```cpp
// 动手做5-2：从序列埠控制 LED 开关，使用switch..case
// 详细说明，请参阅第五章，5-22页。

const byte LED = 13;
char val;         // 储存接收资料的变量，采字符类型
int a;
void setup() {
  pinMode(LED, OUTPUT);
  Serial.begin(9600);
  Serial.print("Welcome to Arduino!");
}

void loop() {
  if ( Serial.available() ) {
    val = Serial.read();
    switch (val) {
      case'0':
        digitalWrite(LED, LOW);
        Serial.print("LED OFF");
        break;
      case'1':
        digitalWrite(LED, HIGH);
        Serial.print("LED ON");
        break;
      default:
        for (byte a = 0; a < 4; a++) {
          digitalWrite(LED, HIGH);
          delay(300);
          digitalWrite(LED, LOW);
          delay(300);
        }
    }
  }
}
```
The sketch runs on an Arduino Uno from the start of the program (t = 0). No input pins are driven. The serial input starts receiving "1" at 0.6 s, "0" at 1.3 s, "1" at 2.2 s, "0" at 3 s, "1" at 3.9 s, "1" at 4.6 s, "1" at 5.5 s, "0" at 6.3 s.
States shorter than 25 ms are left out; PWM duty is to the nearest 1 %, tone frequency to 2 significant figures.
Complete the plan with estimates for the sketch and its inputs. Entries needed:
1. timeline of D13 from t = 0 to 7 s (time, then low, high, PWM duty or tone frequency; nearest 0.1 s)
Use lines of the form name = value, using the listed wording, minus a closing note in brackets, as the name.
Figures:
timeline of D13 from t = 0 to 7 s = 0 s low; 0.6 s high; 1.3 s low; 2.2 s high; 3 s low; 3.9 s high; 6.3 s low
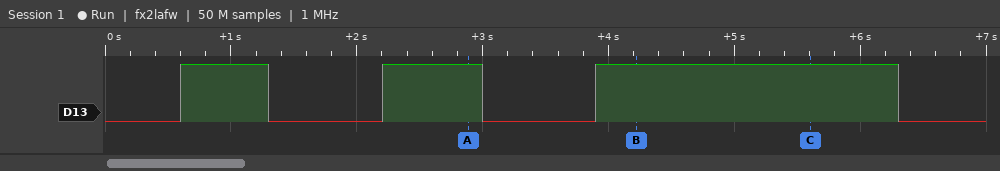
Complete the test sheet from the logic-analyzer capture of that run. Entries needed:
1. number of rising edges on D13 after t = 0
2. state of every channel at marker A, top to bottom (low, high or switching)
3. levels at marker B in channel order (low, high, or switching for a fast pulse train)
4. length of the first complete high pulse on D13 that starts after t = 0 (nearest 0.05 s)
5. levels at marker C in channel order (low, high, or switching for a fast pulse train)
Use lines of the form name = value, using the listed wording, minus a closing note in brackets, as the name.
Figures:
number of rising edges on D13 after t = 0 = 3
state of every channel at marker A, top to bottom = D13 high
levels at marker B in channel order = D13 high
length of the first complete high pulse on D13 that starts after t = 0 = 0.70 s
levels at marker C in channel order = D13 high
